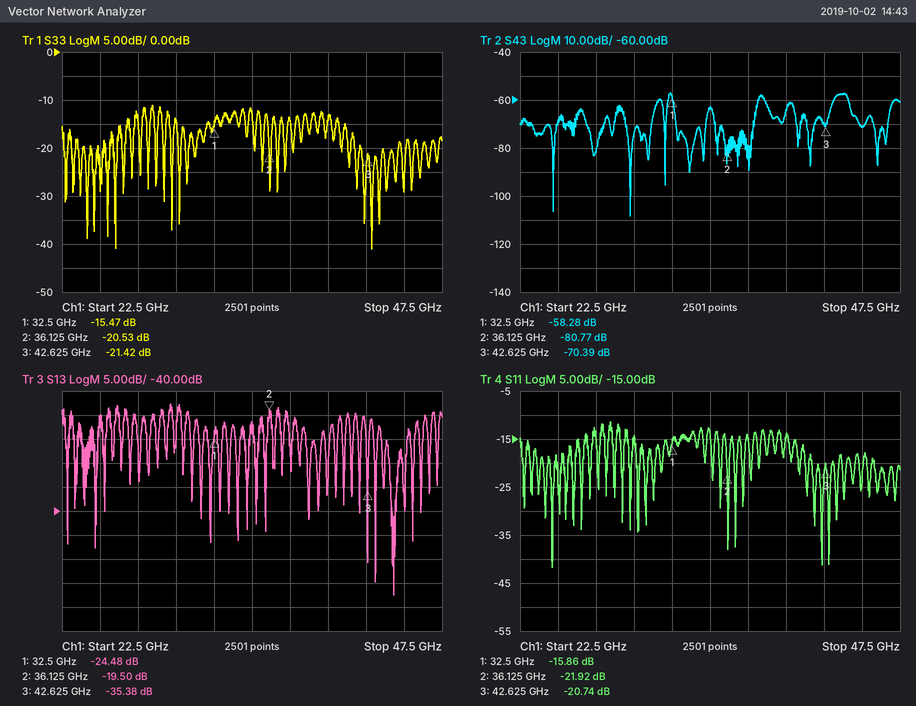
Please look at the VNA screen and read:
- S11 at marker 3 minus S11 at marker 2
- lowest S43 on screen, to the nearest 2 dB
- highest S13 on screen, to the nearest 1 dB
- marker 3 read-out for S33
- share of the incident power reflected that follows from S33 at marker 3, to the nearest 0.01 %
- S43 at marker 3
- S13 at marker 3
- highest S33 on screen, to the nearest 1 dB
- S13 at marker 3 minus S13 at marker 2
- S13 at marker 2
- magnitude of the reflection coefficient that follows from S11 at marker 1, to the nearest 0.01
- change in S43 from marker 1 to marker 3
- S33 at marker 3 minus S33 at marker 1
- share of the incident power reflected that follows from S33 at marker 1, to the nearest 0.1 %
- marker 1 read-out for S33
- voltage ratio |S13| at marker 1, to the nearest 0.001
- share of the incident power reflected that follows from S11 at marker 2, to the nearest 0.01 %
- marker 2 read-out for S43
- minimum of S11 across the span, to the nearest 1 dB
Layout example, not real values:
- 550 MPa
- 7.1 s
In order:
- 1.18 dB
- -108 dB
- -18 dB
- -21.42 dB
- 0.72 %
- -70.39 dB
- -35.38 dB
- -11 dB
- -15.88 dB
- -19.50 dB
- 0.16
- -12.11 dB
- -5.95 dB
- 2.8 %
- -15.47 dB
- 0.060
- 0.64 %
- -80.77 dB
- -42 dB
